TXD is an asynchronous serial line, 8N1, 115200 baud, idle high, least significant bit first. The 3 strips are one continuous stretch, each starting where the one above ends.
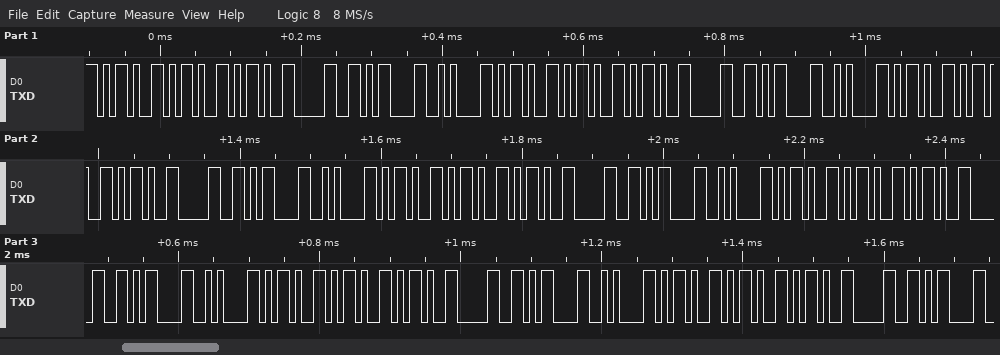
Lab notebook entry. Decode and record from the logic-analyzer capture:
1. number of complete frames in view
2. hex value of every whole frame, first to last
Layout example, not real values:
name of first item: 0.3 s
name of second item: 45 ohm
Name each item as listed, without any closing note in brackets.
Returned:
number of complete frames in view: 41
hex value of every whole frame, first to last: 0x2D 0x2D 0x2D 0x30 0x0D 0x0A 0x2D 0x2D 0x2D 0x30 0x0D 0x0A 0x2D 0x2D 0x2D 0x30 0x0D 0x0A 0x2D 0x2D 0x2D 0x30 0x0D 0x0A 0x2D 0x2D 0x2D 0x30 0x0D 0x0A 0x2D 0x2D 0x2D 0x30 0x0D 0x0A 0x2D 0x2D 0x2D 0x30 0x0D
